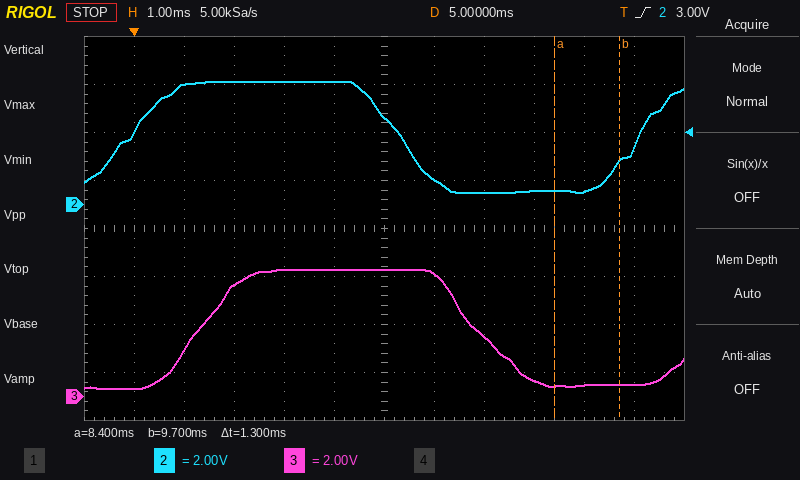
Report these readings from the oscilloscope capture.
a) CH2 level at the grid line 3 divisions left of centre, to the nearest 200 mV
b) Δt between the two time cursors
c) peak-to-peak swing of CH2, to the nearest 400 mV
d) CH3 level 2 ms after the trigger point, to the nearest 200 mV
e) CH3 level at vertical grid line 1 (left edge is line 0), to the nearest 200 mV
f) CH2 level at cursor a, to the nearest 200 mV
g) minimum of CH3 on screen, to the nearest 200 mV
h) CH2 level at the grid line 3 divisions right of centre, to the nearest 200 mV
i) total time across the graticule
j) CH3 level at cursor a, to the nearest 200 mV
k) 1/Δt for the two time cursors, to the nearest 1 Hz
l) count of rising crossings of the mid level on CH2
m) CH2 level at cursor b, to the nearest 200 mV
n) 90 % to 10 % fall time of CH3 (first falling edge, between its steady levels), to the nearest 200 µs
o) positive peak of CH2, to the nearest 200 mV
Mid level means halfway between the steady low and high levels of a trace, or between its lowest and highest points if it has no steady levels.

5.2 V
1.3 ms
4.8 V
4.6 V
400 mV
600 mV
400 mV
600 mV
12 ms
400 mV
769 Hz
2
1.8 V
1.6 ms
5.2 V
